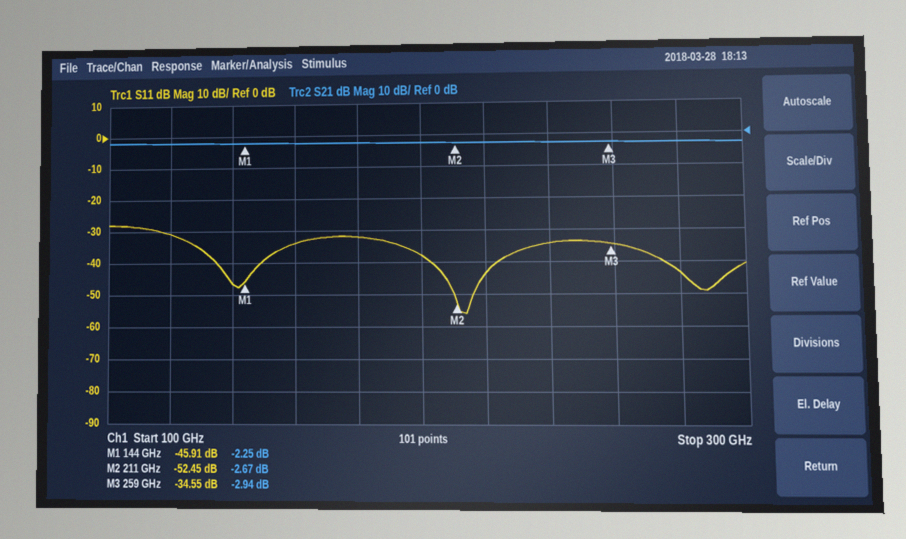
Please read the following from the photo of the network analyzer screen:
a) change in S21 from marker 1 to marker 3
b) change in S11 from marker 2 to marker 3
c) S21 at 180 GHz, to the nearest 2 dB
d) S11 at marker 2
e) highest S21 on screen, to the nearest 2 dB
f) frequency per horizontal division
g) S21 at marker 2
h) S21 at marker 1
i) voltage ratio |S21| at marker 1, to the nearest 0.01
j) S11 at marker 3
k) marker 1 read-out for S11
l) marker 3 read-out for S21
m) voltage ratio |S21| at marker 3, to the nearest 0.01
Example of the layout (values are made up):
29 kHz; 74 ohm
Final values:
-0.69 dB; 17.90 dB; -2 dB; -52.45 dB; -2 dB; 20 GHz; -2.67 dB; -2.25 dB; 0.77; -34.55 dB; -45.91 dB; -2.94 dB; 0.71
